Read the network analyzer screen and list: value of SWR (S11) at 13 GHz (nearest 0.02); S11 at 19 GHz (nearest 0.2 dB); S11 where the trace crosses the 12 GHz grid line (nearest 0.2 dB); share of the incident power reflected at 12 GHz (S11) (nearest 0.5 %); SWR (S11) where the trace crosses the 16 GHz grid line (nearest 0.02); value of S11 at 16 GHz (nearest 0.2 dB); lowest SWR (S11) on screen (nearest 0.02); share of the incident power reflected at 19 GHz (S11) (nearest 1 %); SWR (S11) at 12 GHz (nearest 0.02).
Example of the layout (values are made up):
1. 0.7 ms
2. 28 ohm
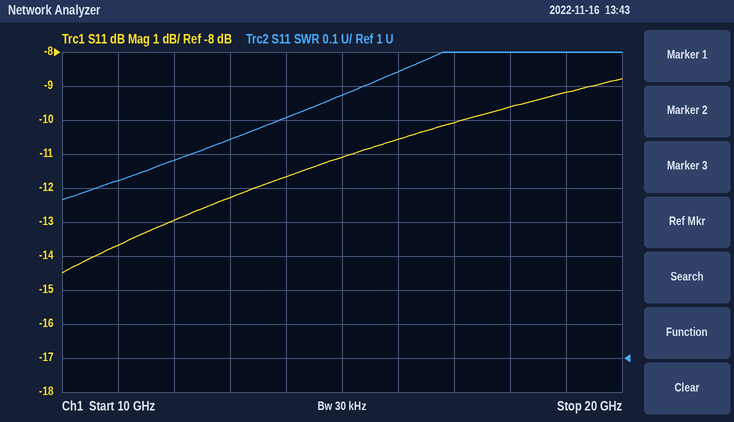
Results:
1. 1.64
2. -9.2 dB
3. -13.0 dB
4. 5.0 %
5. 1.84
6. -10.6 dB
7. 1.46
8. 12 %
9. 1.58
